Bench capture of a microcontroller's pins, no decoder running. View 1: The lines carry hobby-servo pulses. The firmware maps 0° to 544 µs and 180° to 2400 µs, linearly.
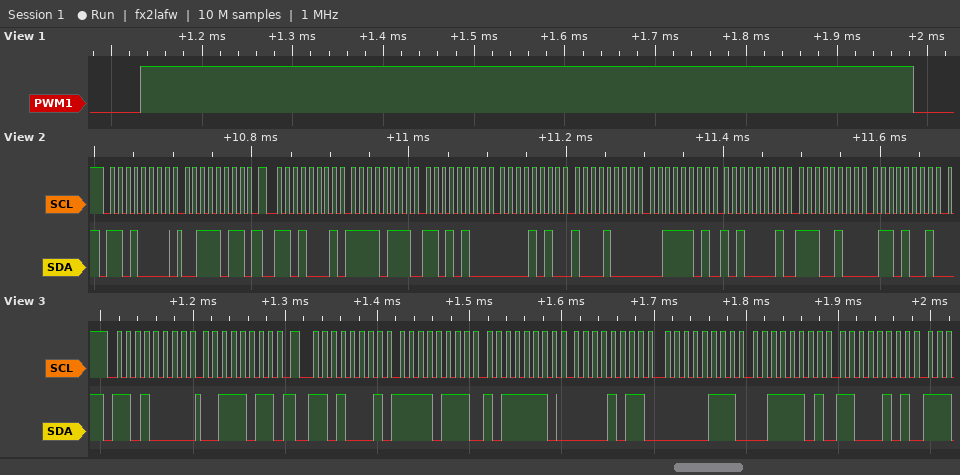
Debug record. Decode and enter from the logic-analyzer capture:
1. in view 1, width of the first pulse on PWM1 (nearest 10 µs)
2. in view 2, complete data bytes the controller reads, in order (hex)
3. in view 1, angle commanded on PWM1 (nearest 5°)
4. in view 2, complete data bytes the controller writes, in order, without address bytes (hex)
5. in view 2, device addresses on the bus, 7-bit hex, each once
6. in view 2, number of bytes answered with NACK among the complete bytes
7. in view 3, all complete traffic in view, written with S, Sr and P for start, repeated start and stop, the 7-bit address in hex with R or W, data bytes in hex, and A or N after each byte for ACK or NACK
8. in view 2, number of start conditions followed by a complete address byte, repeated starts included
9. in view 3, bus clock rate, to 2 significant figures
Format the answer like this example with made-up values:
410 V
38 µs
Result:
850 µs
F7 D4 0A 88 3D A1 E4 69
30°
3B
0x68
0
S 68W A 3B A Sr 68R A F7 A BE A 0B A 07 A 3D A C5 A
2
100 kHz
